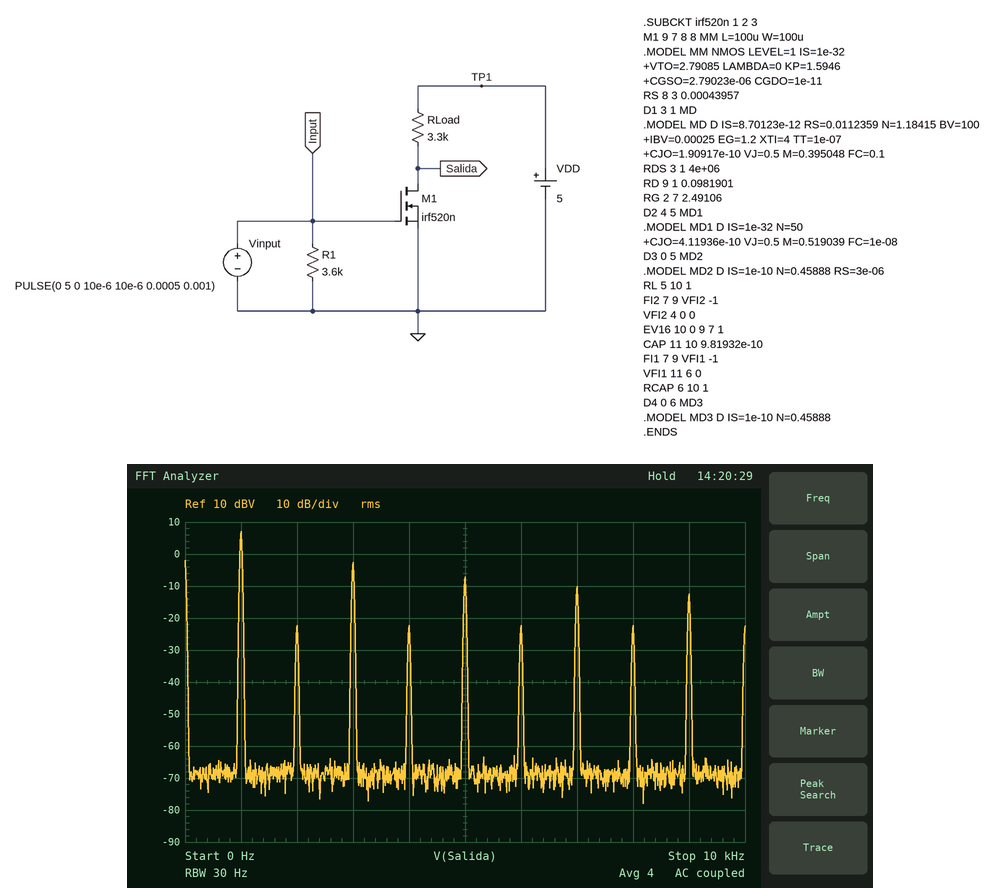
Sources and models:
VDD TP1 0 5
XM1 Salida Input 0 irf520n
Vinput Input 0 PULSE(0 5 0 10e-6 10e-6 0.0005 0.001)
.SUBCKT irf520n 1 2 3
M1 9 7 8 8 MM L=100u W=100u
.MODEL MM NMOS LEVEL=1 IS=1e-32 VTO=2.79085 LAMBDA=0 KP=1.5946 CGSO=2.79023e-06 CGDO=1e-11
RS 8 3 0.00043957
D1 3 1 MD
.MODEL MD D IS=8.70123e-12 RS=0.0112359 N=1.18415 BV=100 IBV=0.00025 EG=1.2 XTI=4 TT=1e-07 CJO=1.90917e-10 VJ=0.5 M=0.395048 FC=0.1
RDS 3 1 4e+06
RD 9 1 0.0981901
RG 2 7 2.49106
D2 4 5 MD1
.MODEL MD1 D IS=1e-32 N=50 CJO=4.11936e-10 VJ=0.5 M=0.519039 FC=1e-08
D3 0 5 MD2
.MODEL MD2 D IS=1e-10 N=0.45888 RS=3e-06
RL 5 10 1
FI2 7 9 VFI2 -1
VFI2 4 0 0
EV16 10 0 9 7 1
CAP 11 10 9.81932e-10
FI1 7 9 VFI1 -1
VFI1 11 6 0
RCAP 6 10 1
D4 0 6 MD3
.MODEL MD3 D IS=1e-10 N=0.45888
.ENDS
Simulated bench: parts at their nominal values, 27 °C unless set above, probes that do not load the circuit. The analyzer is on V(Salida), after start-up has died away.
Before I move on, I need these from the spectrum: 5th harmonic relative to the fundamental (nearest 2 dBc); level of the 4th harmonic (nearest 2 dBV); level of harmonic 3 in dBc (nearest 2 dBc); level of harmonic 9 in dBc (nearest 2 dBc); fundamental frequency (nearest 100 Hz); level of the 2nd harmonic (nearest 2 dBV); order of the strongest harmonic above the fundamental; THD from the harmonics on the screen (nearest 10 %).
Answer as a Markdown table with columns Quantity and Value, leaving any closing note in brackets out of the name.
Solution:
| Quantity | Value |
|---|---|
| 5th harmonic relative to the fundamental | -14 dBc |
| level of the 4th harmonic | -22 dBV |
| level of harmonic 3 in dBc | -10 dBc |
| level of harmonic 9 in dBc | -20 dBc |
| fundamental frequency | 1.0 kHz |
| level of the 2nd harmonic | -22 dBV |
| order of the strongest harmonic above the fundamental | 3 |
| THD from the harmonics on the screen | 40 % |
